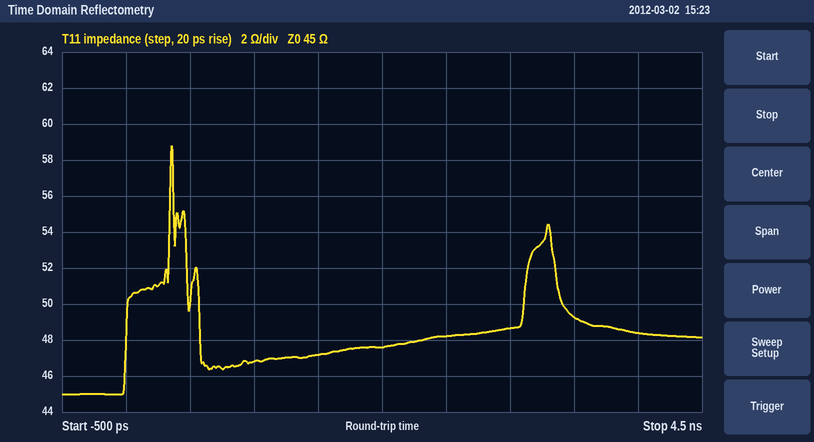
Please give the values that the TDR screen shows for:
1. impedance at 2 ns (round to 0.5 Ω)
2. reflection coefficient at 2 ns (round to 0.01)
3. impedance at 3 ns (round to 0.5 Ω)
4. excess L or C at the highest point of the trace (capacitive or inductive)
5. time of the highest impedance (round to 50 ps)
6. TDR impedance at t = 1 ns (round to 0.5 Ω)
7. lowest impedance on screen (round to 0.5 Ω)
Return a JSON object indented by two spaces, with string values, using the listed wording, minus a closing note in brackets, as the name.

{
  "impedance at 2 ns": "47.5 Ω",
  "reflection coefficient at 2 ns": "+0.03",
  "impedance at 3 ns": "48.5 Ω",
  "excess L or C at the highest point of the trace": "inductive",
  "time of the highest impedance": "350 ps",
  "TDR impedance at t = 1 ns": "47.0 Ω",
  "lowest impedance on screen": "45.0 Ω"
}
